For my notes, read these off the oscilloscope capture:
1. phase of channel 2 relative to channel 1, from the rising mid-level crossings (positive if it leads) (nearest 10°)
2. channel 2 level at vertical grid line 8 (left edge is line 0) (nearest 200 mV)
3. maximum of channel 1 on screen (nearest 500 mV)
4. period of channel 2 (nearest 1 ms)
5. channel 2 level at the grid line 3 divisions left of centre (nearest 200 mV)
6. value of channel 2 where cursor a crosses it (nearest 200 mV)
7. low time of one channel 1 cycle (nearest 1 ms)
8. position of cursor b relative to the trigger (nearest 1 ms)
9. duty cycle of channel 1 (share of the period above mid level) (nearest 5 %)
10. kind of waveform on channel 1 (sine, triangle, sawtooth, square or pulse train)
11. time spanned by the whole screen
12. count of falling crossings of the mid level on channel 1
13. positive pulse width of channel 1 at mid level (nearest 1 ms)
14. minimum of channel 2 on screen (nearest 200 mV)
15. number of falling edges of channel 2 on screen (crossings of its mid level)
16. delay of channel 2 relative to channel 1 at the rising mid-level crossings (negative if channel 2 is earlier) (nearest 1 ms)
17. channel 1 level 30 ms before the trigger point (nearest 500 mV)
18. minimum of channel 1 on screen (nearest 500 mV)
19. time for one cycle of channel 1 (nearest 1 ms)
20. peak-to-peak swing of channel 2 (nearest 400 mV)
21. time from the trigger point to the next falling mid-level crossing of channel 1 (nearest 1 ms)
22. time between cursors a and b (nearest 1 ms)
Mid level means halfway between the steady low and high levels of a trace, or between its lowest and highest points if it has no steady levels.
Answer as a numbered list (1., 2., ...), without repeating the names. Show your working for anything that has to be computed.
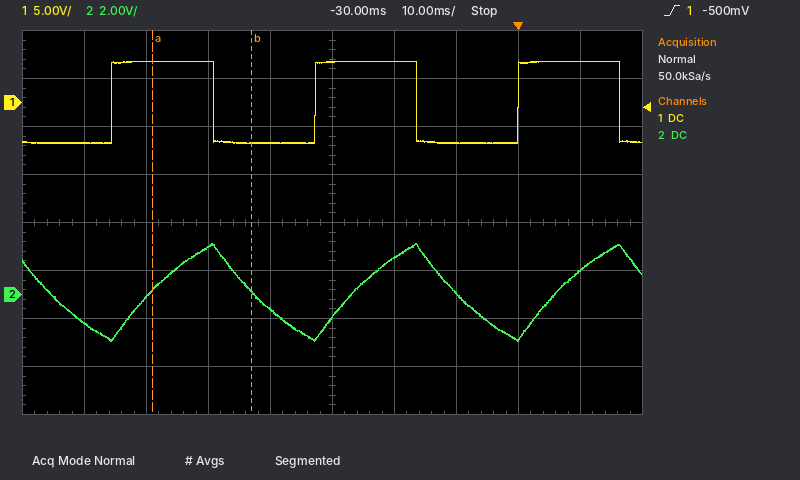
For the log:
1. −360° × (+6 ms) / 33 ms ≈ -65.5°, so -70° to the nearest 10°
2. -1.8 V
3. 4.5 V
4. 33 ms
5. -200 mV
6. 200 mV
7. 16 ms
8. -43 ms
9. 16 ms / 33 ms ≈ 48.5 %, so 50 % to the nearest 5 %
10. square
11. 100 ms
12. 3
13. 16 ms
14. -2.0 V
15. 3
16. +6 ms
17. 4.0 V
18. -4.5 V
19. 33 ms
20. 4.0 V
21. 16 ms
22. 16 ms
